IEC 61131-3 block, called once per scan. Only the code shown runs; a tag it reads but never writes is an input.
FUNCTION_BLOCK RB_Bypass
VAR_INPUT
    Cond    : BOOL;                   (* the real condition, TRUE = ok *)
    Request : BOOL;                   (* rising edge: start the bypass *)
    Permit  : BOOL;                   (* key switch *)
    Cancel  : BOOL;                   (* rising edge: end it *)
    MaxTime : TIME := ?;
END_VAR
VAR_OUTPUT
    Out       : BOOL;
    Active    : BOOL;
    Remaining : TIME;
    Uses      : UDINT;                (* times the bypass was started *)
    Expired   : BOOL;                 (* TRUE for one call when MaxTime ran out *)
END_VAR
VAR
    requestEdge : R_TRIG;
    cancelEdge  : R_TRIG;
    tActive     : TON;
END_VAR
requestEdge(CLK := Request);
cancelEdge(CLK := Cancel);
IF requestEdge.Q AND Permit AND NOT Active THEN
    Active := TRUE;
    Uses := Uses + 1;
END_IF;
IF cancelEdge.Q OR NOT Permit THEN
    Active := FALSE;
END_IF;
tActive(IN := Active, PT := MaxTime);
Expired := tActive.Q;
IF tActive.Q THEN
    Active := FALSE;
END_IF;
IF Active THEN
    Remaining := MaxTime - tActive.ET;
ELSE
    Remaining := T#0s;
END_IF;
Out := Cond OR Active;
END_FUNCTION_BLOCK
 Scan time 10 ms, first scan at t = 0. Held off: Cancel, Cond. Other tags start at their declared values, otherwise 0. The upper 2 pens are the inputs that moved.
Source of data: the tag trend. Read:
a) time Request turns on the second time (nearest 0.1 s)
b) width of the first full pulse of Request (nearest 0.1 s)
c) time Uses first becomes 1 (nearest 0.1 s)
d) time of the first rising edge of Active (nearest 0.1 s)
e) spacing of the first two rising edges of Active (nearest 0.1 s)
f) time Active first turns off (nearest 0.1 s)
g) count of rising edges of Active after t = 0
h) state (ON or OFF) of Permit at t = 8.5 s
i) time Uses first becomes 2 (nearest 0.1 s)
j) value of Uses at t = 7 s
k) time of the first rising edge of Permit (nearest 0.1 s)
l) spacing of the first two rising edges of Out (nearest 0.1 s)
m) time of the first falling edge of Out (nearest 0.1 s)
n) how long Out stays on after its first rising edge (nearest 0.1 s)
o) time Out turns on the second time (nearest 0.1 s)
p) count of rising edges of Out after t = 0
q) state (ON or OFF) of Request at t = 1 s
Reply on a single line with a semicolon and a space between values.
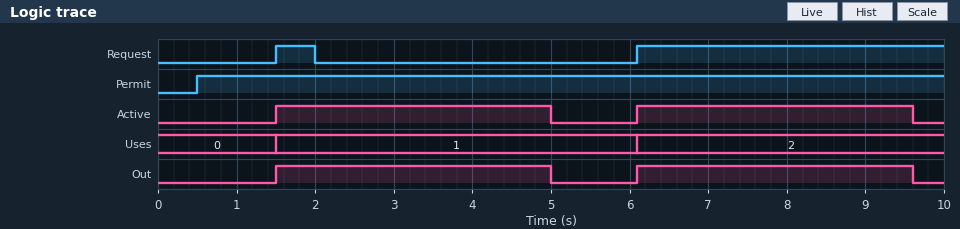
6.1 s; 0.5 s; 1.5 s; 1.5 s; 4.6 s; 5.0 s; 2; ON; 6.1 s; 2; 0.5 s; 4.6 s; 5.0 s; 3.5 s; 6.1 s; 2; OFF
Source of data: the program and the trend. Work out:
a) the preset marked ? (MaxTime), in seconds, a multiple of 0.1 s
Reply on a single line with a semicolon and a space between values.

3.5 s
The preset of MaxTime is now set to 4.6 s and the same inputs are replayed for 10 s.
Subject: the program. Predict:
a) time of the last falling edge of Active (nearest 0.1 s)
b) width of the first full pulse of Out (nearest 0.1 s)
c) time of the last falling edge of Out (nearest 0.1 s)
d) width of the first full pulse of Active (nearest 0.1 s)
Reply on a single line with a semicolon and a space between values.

6.1 s; 4.6 s; 6.1 s; 4.6 s
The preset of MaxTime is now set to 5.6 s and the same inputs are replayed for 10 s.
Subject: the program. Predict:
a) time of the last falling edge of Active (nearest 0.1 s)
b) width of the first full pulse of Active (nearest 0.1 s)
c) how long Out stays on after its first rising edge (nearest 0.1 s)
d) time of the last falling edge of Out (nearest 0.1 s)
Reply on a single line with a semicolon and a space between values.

7.1 s; 5.6 s; 5.6 s; 7.1 s
